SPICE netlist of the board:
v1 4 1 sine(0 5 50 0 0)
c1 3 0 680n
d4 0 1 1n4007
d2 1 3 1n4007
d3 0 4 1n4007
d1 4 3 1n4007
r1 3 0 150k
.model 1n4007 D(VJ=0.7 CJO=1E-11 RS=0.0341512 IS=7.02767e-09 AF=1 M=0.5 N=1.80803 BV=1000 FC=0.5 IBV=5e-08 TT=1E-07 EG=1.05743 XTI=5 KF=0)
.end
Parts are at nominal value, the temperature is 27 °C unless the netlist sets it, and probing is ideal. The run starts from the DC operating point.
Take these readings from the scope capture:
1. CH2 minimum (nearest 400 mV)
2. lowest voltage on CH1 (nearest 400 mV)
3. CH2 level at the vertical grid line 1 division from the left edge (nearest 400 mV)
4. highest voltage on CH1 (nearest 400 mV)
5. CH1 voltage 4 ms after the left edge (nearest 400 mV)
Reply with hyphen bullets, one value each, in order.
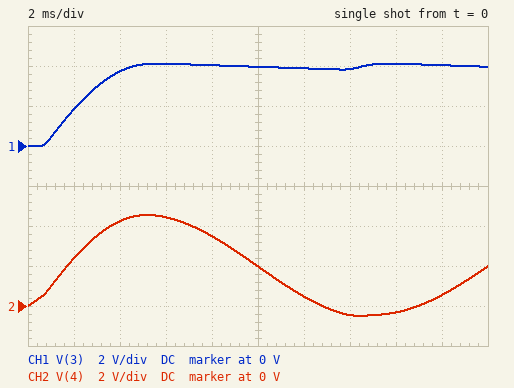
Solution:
- -400 mV
- 0 V
- 2.4 V
- 4.0 V
- 3.6 V
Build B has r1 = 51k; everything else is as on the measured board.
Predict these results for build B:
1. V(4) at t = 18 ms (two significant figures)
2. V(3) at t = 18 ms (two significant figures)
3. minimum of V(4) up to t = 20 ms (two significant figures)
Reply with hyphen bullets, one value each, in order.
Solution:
- 440 mV
- 3.8 V
- -520 mV
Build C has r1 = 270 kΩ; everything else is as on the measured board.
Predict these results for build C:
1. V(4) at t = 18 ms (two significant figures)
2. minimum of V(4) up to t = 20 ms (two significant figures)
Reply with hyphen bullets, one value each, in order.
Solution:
- 580 mV
- -460 mV
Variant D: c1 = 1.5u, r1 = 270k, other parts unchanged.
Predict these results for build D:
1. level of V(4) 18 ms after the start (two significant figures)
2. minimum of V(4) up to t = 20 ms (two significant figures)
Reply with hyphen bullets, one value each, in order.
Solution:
- 570 mV
- -470 mV
